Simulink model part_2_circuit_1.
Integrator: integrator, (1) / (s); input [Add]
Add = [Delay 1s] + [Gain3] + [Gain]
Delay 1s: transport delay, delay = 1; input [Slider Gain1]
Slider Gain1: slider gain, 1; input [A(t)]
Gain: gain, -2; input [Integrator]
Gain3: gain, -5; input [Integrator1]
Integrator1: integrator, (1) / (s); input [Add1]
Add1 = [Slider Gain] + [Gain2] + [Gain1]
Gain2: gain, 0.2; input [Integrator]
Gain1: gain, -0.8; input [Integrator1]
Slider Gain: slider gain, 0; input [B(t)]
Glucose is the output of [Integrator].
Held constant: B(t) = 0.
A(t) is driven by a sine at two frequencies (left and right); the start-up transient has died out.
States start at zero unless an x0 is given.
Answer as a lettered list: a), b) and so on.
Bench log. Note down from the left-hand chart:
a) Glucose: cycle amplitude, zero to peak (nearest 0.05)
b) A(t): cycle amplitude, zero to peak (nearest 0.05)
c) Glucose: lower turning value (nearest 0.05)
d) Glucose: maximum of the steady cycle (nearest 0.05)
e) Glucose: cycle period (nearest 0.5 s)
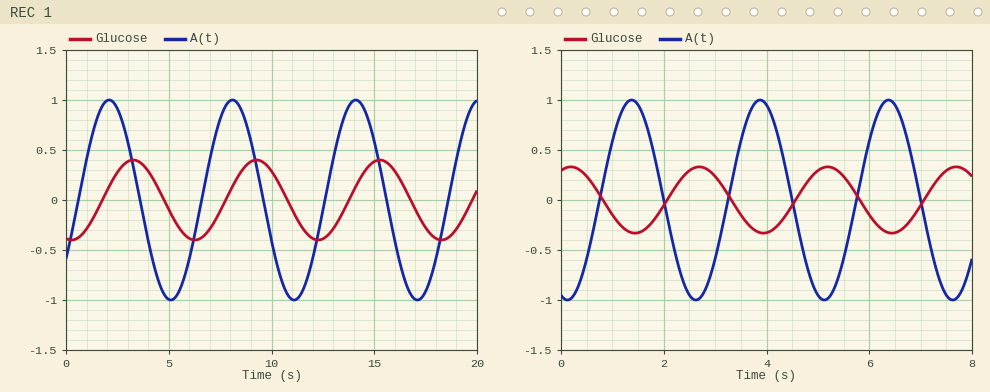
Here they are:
a) 0.40
b) 1.00
c) -0.40
d) 0.40
e) 6.0 s
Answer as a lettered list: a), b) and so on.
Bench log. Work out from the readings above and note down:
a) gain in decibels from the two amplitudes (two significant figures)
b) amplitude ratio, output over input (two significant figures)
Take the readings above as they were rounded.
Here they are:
a) -8.0 dB
b) 0.40
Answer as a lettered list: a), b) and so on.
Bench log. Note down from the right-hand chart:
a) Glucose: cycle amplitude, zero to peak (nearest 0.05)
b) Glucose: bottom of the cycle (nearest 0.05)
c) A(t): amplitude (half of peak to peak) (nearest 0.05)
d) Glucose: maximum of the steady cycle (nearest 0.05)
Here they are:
a) 0.35
b) -0.35
c) 1.00
d) 0.35
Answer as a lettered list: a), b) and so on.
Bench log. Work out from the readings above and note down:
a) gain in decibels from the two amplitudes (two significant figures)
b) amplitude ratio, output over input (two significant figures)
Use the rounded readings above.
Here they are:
a) -9.1 dB
b) 0.35
